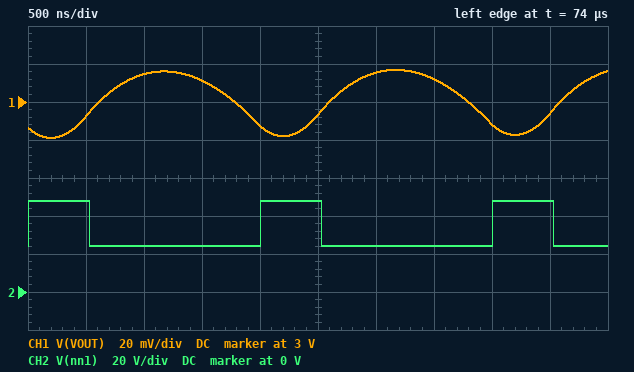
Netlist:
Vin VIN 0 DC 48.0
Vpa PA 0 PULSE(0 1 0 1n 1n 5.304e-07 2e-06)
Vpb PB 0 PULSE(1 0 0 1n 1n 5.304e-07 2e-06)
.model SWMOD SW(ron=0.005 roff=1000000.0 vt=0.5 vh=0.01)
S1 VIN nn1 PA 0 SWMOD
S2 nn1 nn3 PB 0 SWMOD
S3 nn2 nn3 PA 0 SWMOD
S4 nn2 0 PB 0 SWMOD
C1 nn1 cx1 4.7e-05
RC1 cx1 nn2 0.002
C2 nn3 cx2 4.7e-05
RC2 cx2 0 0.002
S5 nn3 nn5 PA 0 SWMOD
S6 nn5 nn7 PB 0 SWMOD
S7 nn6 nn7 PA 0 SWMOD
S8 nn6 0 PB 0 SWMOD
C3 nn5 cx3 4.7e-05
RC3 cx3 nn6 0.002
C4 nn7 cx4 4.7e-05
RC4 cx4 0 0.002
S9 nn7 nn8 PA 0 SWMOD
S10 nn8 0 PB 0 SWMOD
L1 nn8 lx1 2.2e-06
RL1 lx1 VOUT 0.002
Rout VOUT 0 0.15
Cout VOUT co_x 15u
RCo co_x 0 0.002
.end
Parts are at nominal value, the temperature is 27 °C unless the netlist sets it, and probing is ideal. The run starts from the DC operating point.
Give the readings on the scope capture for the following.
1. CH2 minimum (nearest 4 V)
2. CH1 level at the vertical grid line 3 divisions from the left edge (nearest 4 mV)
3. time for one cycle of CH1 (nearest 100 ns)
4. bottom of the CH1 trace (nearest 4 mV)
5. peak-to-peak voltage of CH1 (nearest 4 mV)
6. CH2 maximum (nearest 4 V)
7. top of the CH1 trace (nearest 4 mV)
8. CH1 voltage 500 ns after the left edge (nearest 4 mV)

24 V
3.012 V
2.0 µs
2.980 V
36 mV
48 V
3.016 V
2.992 V
